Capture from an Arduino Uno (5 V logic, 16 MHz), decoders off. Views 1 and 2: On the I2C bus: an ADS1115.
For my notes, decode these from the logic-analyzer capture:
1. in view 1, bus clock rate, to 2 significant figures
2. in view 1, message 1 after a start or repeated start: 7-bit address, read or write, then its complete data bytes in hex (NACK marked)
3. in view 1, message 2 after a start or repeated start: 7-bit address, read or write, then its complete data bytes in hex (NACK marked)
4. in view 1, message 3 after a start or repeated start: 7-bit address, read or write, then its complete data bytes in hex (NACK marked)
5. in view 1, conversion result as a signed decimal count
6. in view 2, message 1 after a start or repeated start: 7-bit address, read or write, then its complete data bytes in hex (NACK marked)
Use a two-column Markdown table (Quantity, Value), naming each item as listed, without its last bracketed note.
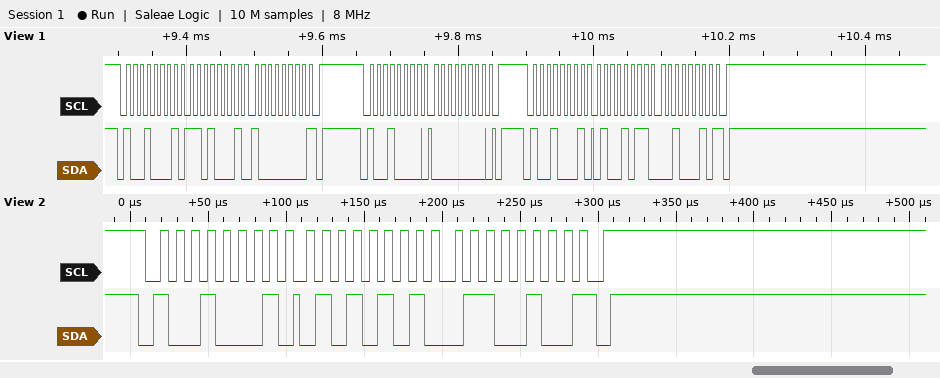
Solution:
| Quantity | Value |
|---|---|
| in view 1, bus clock rate, to 2 significant figures | 100 kHz |
| in view 1, message 1 after a start or repeated start: 7-bit address, read or write, then its complete data bytes in hex | 0x48 read: D1 80 NACK |
| in view 1, message 2 after a start or repeated start: 7-bit address, read or write, then its complete data bytes in hex | 0x48 write: 00 |
| in view 1, message 3 after a start or repeated start: 7-bit address, read or write, then its complete data bytes in hex | 0x48 read: 4B 22 NACK |
| in view 1, conversion result as a signed decimal count | 19234 |
| in view 2, message 1 after a start or repeated start: 7-bit address, read or write, then its complete data bytes in hex | 0x48 read: 55 64 NACK |
